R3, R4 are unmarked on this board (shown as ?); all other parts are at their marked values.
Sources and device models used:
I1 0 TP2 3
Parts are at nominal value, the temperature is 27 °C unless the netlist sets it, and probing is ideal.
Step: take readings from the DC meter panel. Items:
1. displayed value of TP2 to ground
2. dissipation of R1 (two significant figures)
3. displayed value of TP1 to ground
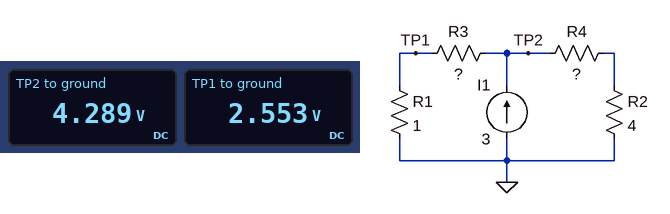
4.289 V
6.5 W
2.553 V
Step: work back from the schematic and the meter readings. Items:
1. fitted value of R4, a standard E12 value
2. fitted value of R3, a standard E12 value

5.6 Ω
0.68 Ω
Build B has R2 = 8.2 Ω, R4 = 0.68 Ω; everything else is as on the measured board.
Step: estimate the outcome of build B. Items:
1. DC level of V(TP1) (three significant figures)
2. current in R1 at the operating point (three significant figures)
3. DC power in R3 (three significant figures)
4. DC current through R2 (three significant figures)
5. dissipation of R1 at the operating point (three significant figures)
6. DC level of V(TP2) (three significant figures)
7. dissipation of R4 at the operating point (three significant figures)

2.52 V
2.52 A
4.33 W
477 mA
6.36 W
4.24 V
155 mW
